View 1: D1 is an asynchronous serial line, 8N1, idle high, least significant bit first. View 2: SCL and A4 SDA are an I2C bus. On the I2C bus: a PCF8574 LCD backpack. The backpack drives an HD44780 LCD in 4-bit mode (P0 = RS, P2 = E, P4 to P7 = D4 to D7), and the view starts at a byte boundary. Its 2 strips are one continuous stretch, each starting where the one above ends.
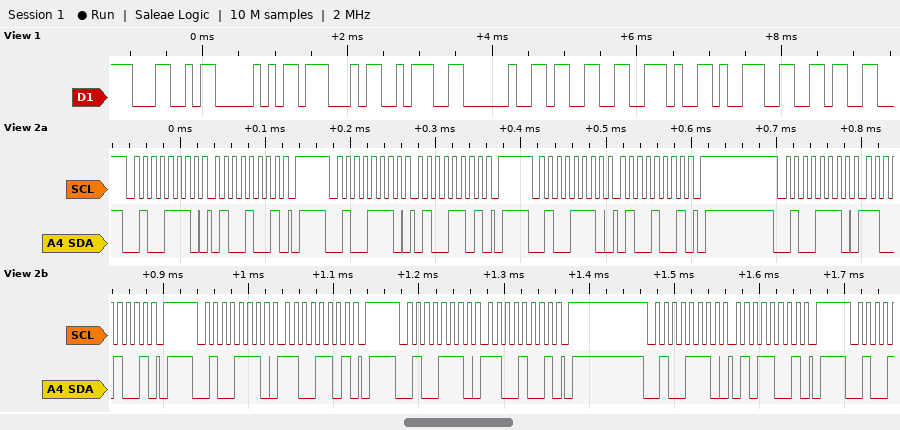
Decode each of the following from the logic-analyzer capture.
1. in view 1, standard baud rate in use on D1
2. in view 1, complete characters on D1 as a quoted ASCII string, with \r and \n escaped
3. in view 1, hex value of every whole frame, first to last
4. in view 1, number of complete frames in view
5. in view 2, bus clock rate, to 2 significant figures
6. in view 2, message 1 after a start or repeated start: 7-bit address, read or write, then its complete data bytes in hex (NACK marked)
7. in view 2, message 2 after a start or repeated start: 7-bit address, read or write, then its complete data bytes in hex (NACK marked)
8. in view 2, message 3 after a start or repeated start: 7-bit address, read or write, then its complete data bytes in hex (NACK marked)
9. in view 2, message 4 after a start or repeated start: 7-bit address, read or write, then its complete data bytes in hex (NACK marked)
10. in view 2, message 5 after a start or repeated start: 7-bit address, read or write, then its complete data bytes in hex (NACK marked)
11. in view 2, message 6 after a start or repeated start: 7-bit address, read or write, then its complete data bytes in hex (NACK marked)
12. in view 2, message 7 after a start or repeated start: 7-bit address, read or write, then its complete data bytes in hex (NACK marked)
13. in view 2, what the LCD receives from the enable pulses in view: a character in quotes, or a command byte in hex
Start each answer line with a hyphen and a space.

- 9600 baud
- "LPG: 3.96"
- 4C 50 47 3A 20 33 2E 39 36
- 9
- 100 kHz
- 0x27 write: 49
- 0x27 write: 4D
- 0x27 write: 49
- 0x27 write: C9
- 0x27 write: CD
- 0x27 write: C9
- 0x27 write: 59
- 'L'
